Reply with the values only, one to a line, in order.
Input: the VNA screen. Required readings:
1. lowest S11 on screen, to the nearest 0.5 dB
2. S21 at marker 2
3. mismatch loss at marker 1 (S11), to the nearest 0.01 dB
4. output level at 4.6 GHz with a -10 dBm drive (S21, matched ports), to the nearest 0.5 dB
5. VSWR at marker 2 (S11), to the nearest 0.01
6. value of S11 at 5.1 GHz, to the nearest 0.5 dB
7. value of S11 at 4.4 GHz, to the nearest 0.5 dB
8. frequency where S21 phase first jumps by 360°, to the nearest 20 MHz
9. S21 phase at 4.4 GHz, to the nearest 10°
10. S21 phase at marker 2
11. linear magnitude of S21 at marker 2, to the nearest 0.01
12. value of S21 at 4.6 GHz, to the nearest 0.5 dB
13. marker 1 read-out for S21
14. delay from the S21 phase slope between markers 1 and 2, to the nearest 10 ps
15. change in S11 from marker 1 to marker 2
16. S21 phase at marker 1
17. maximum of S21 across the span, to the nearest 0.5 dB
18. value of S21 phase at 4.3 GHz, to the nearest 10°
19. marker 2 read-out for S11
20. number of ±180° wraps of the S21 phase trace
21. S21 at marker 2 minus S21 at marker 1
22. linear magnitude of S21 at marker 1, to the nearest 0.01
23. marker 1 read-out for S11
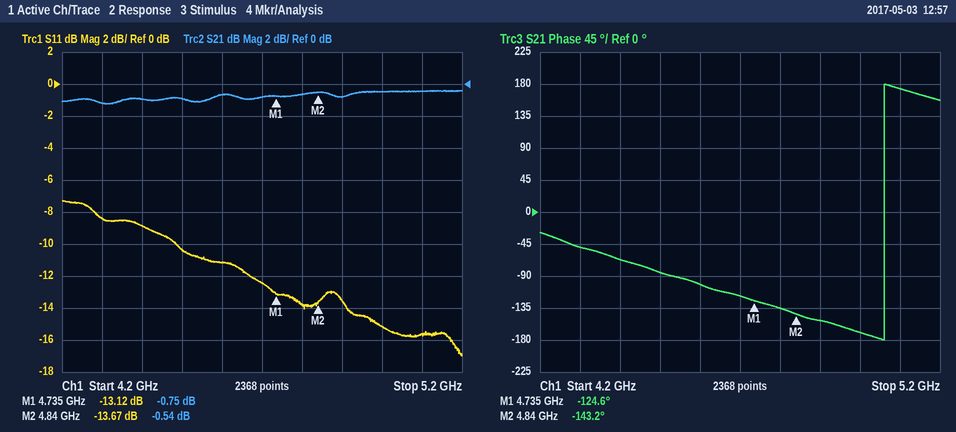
-17.0 dB
-0.54 dB
0.22 dB
-10.5 dBm
1.52
-15.5 dB
-9.0 dB
5.06 GHz
-70°
-143.2°
0.94
-0.5 dB
-0.75 dB
490 ps
-0.55 dB
-124.6°
-0.5 dB
-50°
-13.67 dB
1
0.21 dB
0.92
-13.12 dB
